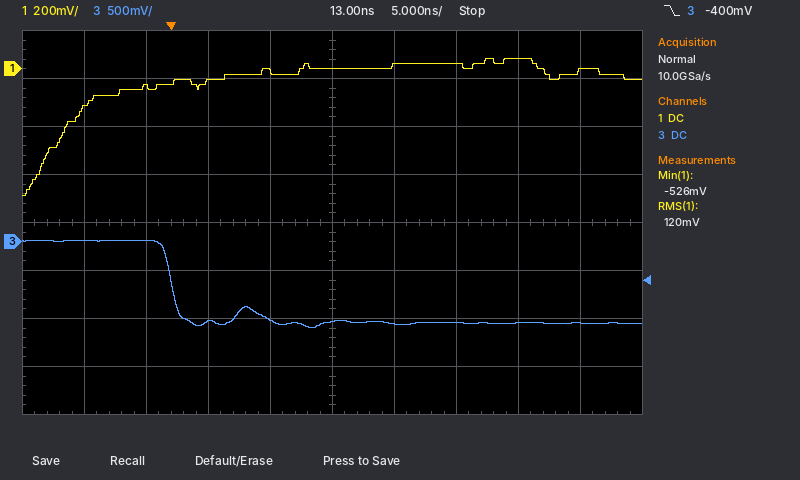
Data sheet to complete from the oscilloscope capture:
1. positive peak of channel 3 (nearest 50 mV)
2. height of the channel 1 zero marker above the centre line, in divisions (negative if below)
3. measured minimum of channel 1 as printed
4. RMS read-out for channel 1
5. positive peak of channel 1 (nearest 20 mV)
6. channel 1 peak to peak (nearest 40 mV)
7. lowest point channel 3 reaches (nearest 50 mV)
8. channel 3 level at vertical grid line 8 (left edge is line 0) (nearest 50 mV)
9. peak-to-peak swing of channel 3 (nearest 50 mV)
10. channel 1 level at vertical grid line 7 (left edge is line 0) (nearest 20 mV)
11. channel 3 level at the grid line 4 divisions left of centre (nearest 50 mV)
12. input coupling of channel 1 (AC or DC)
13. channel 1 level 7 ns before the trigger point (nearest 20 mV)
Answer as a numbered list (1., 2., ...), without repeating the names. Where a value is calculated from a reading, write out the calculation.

1. 0 mV
2. +3.2 div
3. -526 mV
4. 120 mV
5. 40 mV
6. 560 mV
7. -900 mV
8. -850 mV
9. 0 mV − (-900 mV) = 900 mV
10. 20 mV
11. 0 mV
12. DC
13. -160 mV
